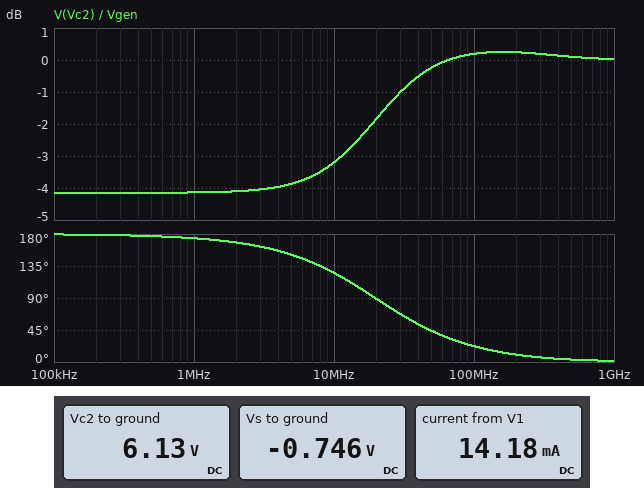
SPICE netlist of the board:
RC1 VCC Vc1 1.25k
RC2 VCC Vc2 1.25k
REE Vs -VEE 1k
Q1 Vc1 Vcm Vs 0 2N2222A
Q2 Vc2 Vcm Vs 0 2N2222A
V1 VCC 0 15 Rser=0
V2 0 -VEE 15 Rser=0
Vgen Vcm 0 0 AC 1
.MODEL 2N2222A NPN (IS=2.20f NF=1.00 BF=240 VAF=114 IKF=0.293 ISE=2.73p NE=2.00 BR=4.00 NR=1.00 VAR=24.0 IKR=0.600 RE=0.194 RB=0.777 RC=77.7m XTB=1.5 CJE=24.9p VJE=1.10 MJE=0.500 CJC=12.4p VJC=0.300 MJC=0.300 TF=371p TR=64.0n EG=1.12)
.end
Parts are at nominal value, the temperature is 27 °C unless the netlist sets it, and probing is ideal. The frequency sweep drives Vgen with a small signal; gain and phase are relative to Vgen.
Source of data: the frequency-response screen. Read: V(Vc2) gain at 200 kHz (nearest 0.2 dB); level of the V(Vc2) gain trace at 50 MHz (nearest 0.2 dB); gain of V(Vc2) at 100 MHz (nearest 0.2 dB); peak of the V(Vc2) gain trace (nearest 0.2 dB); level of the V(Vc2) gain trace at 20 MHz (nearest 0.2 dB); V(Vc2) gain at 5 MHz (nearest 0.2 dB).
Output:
-4.2 dB
-0.2 dB
0.2 dB
0.2 dB
-1.8 dB
-3.8 dB
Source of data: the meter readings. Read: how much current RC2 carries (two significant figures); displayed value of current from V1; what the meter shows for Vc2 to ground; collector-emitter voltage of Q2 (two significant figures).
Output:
7.1 mA
14.18 mA
6.13 V
6.9 V
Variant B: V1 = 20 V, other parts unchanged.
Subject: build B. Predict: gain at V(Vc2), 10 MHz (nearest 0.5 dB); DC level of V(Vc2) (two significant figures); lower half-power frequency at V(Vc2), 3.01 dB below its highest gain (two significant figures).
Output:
-3.5 dB
11 V
15 MHz
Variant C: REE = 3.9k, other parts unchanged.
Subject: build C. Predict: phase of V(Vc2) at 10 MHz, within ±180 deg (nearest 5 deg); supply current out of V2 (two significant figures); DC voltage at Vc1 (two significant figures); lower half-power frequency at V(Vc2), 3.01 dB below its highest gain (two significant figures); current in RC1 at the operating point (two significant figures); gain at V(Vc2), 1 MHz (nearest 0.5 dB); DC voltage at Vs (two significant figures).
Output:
100 deg
3.7 mA
13 V
29 MHz
1.8 mA
-16.0 dB
-710 mV
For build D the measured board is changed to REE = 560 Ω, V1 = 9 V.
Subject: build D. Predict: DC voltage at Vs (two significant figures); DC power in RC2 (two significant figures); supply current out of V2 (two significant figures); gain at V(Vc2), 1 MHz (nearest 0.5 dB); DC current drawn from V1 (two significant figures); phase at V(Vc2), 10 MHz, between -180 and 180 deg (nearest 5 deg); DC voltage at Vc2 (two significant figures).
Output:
-790 mV
76 mW
25 mA
0 dB
16 mA
0 deg
-770 mV
